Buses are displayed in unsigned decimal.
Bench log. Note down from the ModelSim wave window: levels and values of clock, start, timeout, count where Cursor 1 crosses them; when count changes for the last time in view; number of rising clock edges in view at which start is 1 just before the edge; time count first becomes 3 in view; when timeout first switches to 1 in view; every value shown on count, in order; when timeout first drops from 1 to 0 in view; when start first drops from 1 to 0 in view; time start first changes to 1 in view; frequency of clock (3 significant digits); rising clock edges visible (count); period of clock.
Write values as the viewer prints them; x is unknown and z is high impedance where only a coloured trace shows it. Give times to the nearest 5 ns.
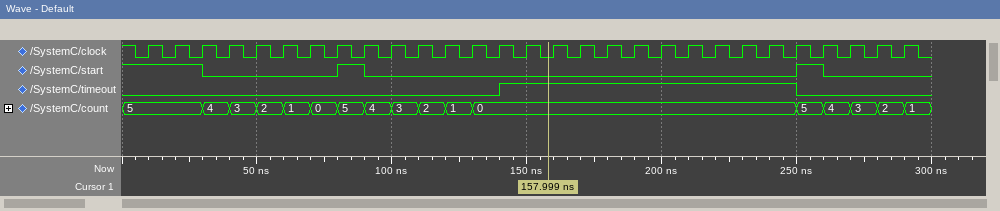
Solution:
clock=0, start=0, timeout=1, count=0
290 ns
5
40 ns
140 ns
5, 4, 3, 2, 1, 0, 5, 4, 3, 2, 1, 0, 5, 4, 3, 2, 1
250 ns
30 ns
80 ns
100 MHz
29
10 ns
